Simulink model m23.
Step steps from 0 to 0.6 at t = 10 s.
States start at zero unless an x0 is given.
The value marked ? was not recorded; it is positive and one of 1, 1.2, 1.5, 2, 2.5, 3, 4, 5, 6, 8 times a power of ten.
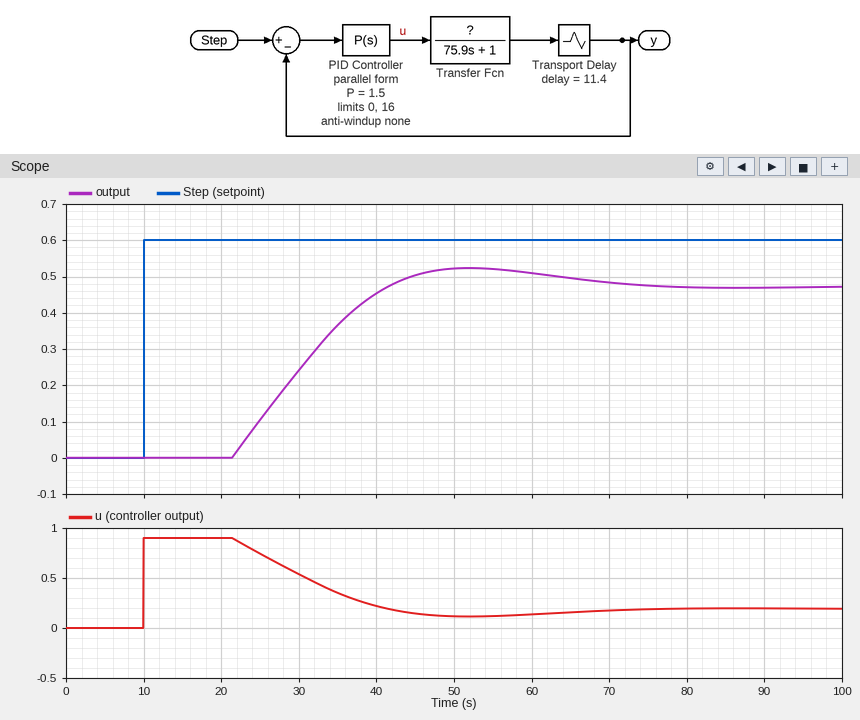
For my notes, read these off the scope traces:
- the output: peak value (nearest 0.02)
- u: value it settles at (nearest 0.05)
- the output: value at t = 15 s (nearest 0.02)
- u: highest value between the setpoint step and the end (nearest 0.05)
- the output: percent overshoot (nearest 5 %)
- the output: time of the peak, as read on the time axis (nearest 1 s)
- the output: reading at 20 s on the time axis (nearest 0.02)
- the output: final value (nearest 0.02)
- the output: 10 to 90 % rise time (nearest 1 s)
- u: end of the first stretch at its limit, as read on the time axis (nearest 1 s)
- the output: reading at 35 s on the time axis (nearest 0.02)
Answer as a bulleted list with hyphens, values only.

- 0.52
- 0.20
- 0.00
- 0.90
- 10 %
- 52 s
- 0.00
- 0.48
- 15 s
- 22 s
- 0.36
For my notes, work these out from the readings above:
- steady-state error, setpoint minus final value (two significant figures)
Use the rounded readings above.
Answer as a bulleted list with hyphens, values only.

- 0.12
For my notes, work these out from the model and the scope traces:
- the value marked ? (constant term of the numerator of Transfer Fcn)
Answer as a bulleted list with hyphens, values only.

- 2.5
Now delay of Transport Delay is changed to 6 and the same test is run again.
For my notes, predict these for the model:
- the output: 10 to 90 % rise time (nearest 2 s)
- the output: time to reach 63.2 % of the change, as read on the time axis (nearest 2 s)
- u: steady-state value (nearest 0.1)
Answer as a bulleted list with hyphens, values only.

- 22 s
- 28 s
- 0.2
